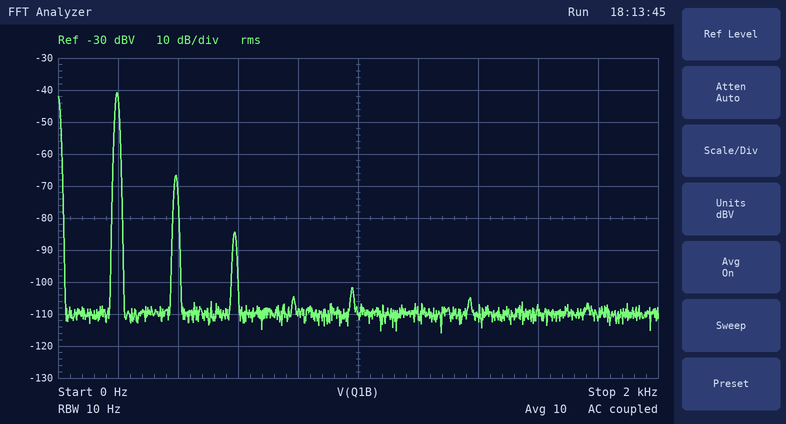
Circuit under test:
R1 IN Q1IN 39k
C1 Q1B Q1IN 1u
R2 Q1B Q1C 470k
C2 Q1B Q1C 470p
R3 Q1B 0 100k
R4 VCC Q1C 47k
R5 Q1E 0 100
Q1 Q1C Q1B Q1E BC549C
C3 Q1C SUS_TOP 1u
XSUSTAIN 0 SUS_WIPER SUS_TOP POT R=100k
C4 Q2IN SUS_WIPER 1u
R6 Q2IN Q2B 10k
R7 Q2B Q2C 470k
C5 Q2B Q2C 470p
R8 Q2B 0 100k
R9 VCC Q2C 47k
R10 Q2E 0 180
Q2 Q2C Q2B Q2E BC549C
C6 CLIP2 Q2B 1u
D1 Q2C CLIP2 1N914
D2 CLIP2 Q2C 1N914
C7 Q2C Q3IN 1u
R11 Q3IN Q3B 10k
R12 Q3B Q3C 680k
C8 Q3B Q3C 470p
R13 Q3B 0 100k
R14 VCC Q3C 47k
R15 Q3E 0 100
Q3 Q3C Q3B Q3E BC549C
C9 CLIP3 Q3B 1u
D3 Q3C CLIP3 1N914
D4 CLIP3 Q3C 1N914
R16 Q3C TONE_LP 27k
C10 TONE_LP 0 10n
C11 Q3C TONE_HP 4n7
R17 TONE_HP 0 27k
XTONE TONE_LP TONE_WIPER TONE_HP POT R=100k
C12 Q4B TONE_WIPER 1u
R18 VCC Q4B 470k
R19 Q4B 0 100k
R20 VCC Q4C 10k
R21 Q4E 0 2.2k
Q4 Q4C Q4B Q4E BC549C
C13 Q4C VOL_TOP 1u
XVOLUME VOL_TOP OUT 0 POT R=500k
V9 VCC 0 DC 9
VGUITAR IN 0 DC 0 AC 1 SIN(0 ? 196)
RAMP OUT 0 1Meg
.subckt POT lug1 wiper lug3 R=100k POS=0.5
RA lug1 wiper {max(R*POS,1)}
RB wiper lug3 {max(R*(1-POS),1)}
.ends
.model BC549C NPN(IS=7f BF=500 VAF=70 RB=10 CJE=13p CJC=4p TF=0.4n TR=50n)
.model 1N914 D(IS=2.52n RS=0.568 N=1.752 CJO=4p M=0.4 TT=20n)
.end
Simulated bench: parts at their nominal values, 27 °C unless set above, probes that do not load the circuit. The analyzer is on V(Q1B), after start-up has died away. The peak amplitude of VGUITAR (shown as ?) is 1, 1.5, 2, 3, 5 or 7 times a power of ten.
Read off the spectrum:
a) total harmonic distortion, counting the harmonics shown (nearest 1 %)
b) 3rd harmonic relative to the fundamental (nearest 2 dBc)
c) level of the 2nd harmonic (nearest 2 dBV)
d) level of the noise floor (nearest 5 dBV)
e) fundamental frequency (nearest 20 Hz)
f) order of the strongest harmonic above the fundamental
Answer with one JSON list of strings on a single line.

["5 %", "-44 dBc", "-66 dBV", "-110 dBV", "200 Hz", "2"]
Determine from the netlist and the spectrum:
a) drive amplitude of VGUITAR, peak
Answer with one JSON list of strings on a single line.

["100 mV"]
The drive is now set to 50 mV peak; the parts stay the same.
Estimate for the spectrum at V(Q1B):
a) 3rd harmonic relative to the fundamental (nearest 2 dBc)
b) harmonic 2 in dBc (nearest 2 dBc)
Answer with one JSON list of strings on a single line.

["-48 dBc", "-32 dBc"]
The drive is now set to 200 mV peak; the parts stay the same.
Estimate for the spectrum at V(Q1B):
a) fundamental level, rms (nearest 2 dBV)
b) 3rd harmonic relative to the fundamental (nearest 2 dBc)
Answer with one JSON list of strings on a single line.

["-34 dBV", "-32 dBc"]
